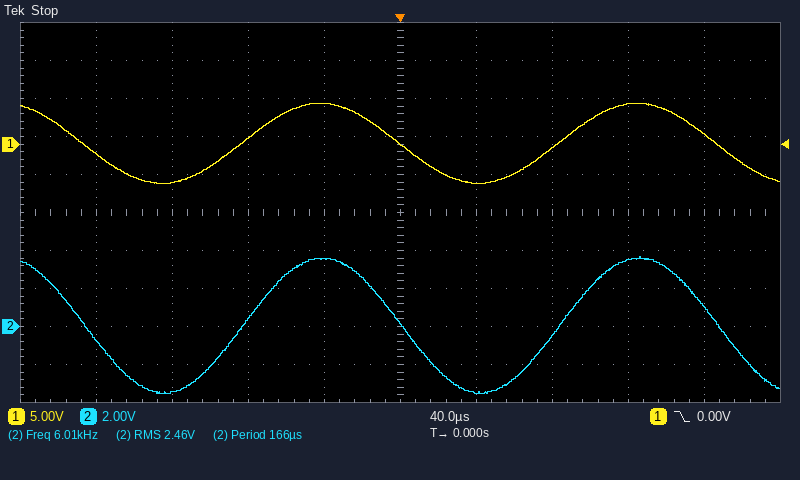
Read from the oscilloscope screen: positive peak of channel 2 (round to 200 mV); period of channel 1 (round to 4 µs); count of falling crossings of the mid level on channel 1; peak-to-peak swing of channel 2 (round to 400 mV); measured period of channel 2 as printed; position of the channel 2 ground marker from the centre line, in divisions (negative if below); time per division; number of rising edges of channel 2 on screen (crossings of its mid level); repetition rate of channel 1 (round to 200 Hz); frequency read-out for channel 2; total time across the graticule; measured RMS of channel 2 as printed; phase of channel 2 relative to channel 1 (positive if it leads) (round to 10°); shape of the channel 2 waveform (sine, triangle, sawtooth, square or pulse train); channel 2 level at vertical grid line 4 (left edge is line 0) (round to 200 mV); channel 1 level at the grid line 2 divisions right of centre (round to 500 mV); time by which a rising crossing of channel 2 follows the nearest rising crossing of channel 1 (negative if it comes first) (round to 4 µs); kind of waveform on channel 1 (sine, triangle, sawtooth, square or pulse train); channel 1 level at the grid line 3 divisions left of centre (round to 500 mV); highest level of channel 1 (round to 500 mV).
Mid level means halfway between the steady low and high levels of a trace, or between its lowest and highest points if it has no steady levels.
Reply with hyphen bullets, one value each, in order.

- 3.6 V
- 168 µs
- 3
- 7.2 V
- 166 µs
- -3.0 div
- 40 µs
- 2
- 6.0 kHz
- 6.01 kHz
- 400 µs
- 2.46 V
- 0°
- sine
- 3.6 V
- -500 mV
- 0 µs
- sine
- -5.0 V
- 5.5 V
